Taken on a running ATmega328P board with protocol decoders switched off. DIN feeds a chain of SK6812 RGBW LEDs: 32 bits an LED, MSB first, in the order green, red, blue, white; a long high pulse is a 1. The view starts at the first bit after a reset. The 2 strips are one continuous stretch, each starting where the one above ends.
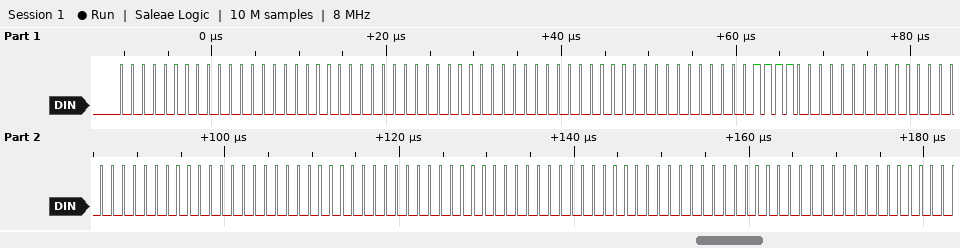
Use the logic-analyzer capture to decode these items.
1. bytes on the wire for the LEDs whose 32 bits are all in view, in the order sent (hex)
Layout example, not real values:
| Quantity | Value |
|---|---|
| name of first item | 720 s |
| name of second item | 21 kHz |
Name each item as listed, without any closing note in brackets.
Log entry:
| Quantity | Value |
|---|---|
| bytes on the wire for the LEDs whose 32 bits are all in view, in the order sent | 00 00 00 00 00 00 00 3C 00 00 00 00 00 00 00 00 |
